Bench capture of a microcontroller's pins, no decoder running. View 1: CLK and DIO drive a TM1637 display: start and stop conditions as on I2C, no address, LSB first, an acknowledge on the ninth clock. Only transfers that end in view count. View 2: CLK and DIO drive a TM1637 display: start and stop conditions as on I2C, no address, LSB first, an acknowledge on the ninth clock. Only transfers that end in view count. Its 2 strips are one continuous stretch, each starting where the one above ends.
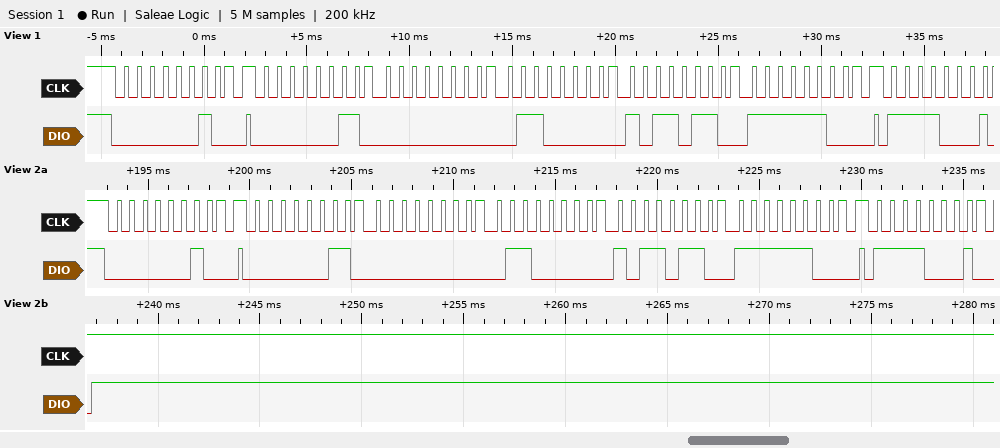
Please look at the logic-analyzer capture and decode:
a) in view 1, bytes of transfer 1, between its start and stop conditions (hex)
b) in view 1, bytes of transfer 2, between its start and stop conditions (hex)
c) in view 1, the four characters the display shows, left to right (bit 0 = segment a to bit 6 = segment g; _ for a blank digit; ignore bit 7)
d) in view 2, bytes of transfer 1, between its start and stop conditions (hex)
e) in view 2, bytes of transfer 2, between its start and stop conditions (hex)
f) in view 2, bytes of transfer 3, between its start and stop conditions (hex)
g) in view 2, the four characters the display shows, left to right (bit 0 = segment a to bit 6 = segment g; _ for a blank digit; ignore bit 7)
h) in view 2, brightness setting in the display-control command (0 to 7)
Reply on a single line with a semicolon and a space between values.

40; C0 00 06 6D 3F; _150; 40; C0 00 06 6D 3F; 8F; _150; 7
